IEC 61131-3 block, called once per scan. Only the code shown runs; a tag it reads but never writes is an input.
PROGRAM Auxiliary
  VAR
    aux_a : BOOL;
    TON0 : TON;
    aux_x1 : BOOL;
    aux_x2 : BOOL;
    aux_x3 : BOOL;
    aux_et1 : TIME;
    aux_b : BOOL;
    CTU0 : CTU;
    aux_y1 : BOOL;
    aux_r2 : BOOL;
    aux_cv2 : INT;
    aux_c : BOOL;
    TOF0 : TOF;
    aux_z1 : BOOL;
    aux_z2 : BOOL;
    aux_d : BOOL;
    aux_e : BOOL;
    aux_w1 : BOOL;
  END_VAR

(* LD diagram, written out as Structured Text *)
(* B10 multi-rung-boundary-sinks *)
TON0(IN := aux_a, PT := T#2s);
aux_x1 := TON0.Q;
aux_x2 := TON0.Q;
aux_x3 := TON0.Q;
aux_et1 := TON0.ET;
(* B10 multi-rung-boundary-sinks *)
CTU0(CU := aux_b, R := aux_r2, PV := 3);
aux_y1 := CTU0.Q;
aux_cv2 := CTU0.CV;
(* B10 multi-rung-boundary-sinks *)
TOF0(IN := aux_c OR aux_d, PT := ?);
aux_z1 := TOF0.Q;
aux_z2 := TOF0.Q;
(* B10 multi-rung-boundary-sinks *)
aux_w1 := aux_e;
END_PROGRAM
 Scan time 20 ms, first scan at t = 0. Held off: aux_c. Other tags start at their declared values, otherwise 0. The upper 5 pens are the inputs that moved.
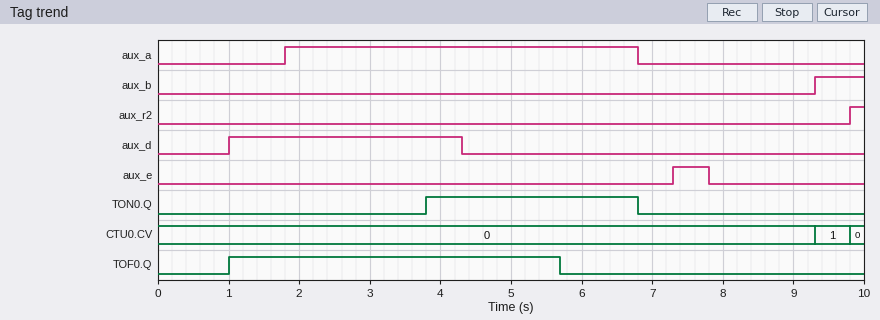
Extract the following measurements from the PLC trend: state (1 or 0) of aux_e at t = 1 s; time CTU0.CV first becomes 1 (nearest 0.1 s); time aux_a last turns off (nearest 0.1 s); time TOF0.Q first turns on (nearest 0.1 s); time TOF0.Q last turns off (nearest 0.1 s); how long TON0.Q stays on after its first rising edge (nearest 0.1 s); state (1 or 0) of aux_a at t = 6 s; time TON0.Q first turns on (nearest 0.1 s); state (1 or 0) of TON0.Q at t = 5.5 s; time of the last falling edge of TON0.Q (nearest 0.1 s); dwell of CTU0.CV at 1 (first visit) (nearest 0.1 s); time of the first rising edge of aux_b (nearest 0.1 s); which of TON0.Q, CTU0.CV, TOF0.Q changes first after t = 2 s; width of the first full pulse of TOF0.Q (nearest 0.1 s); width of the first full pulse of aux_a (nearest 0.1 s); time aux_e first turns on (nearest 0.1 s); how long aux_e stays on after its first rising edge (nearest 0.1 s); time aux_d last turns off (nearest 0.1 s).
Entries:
0
9.3 s
6.8 s
1.0 s
5.7 s
3.0 s
1
3.8 s
1
6.8 s
0.5 s
9.3 s
TON0.Q
4.7 s
5.0 s
7.3 s
0.5 s
4.3 s
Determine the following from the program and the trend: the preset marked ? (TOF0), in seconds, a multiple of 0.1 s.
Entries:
1.4 s
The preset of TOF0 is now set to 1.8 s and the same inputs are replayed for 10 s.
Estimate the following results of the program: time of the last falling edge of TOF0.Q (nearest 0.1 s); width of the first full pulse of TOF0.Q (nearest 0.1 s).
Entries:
6.1 s
5.1 s
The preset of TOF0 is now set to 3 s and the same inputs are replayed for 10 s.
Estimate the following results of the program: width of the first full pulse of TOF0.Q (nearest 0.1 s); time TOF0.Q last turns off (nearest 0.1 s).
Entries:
6.3 s
7.3 s
